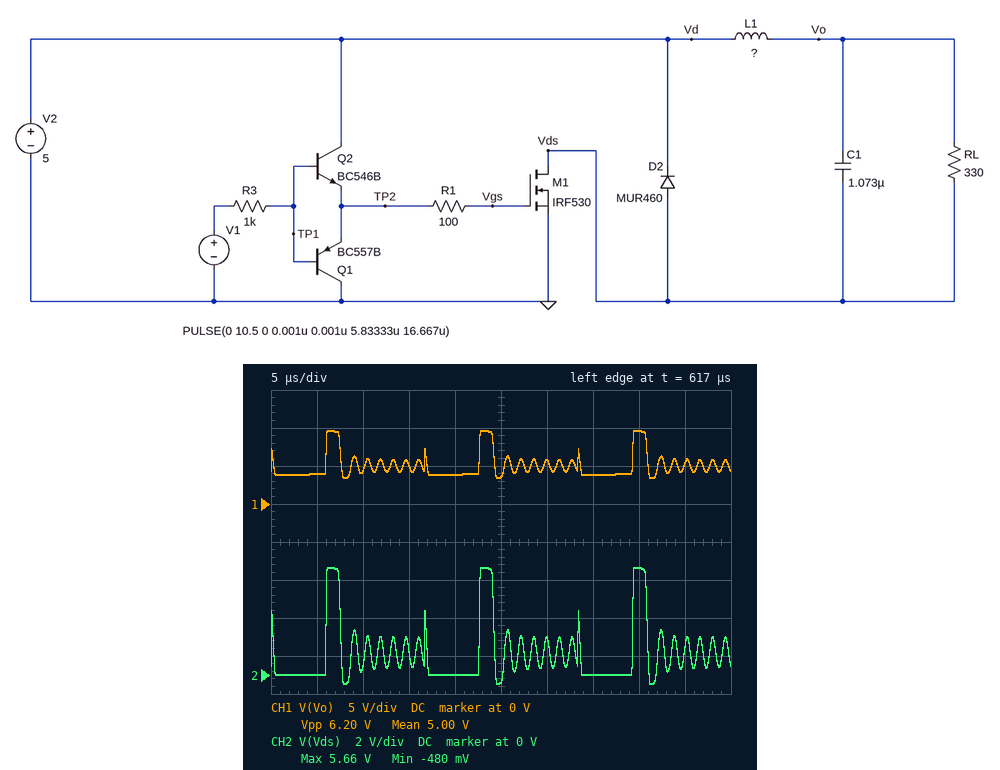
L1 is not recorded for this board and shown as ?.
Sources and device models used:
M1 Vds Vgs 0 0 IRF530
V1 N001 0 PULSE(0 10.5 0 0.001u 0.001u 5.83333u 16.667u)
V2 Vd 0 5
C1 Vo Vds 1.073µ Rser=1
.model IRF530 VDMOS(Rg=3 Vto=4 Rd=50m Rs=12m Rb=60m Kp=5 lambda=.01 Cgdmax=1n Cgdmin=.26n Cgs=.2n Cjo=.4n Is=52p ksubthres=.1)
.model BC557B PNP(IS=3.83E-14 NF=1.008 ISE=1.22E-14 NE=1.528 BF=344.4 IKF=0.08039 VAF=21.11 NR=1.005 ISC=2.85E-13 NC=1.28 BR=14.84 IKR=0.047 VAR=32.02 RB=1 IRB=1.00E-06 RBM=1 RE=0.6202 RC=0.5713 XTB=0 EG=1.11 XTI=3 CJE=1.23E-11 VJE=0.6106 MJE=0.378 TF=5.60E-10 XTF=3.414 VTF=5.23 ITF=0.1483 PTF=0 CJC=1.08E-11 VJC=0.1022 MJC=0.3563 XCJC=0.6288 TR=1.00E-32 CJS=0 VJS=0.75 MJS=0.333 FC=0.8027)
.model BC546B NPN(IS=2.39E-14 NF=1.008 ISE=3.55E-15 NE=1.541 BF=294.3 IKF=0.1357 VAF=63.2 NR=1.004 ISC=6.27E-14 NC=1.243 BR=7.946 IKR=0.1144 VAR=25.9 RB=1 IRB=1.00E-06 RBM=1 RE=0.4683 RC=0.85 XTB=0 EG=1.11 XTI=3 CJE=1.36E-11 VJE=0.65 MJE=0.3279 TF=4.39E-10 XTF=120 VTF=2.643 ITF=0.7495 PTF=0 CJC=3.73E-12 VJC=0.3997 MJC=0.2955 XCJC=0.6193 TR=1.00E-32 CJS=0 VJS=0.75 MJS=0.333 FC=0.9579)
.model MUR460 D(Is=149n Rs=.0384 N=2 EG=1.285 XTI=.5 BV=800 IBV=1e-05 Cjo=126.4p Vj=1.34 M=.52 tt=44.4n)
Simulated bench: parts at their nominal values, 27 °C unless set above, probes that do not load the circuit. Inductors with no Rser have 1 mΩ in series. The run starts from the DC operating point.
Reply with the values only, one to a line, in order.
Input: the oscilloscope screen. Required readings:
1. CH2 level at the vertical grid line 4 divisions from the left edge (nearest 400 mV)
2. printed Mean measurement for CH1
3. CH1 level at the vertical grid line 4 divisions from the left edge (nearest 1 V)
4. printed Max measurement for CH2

0 V
5.00 V
4 V
5.66 V
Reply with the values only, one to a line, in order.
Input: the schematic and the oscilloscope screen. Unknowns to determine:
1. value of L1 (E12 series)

100 µH
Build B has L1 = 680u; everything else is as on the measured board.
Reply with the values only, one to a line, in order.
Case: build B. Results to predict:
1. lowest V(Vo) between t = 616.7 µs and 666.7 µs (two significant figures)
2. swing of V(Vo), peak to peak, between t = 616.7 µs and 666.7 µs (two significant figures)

2.3 V
5.7 V
